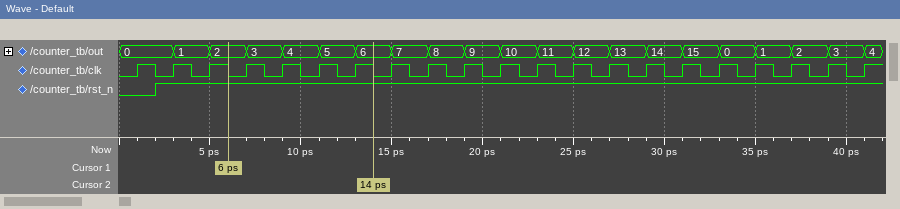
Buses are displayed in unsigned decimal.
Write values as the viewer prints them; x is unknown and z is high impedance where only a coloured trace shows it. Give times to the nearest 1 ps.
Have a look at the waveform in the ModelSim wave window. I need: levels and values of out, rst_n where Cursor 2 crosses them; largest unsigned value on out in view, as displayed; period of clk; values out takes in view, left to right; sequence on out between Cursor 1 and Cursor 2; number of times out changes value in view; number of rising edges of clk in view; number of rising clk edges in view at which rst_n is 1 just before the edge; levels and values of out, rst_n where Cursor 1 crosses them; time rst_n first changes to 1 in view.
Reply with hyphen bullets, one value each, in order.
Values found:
- out=6, rst_n=1
- 15
- 2 ps
- 0, 1, 2, 3, 4, 5, 6, 7, 8, 9, 10, 11, 12, 13, 14, 15, 0, 1, 2, 3, 4
- 2, 3, 4, 5, 6
- 20
- 21
- 20
- out=2, rst_n=1
- 2 ps
